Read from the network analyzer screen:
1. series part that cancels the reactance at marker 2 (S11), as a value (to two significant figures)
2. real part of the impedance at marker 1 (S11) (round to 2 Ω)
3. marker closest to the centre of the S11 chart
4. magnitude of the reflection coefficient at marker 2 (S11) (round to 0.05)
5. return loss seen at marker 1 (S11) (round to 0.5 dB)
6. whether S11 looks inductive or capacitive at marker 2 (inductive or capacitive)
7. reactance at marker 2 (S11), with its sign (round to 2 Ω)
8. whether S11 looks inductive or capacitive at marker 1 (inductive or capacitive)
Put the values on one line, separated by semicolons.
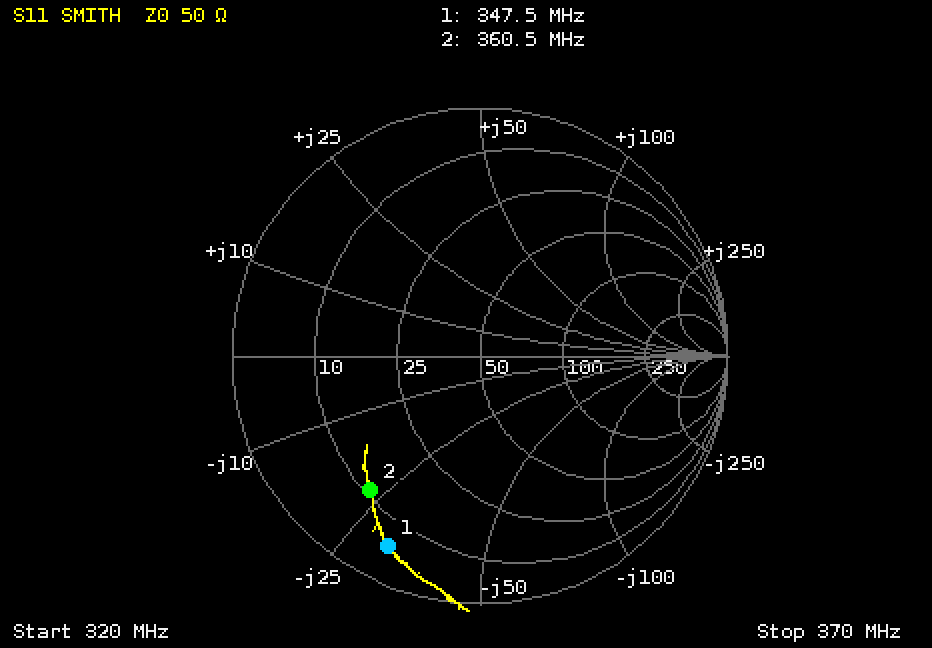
10 nH; 6 Ω; marker 2; 0.70; 1.5 dB; capacitive; -22 Ω; capacitive
